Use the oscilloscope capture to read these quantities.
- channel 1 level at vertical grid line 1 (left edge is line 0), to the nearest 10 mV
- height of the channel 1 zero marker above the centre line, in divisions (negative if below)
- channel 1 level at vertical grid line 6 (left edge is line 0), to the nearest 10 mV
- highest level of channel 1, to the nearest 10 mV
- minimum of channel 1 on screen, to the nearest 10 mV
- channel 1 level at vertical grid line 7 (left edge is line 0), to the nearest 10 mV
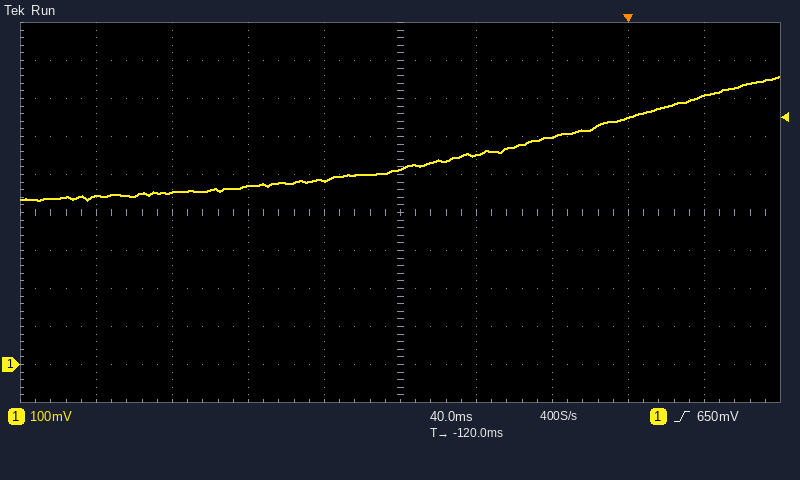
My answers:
440 mV
-4.0 div
550 mV
760 mV
430 mV
600 mV
